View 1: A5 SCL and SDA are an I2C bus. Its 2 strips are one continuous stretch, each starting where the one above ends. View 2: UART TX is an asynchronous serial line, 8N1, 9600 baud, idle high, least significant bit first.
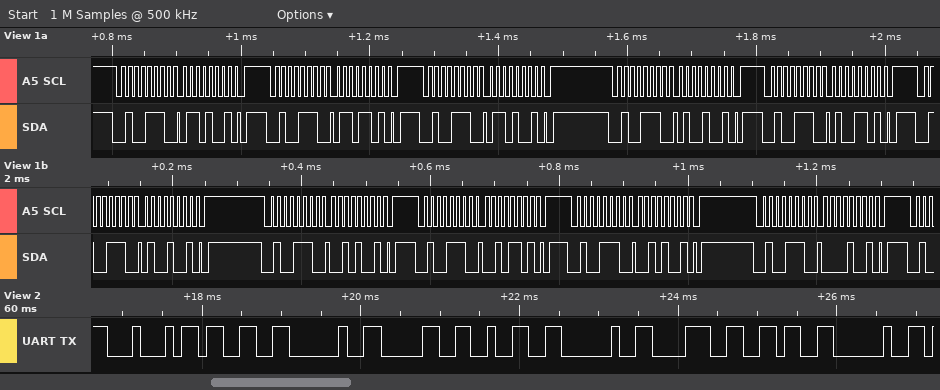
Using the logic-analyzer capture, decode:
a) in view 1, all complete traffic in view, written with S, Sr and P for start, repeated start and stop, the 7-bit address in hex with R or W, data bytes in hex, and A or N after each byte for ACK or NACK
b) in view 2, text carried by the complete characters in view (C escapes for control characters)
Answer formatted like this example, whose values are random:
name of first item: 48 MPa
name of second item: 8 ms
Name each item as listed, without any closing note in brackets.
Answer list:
in view 1, all complete traffic in view, written with S, Sr and P for start, repeated start and stop, the 7-bit address in hex with R or W, data bytes in hex, and A or N after each byte for ACK or NACK: S 27W A 69 A P S 27W A 6D A P S 27W A 69 A P S 27W A 49 A P S 27W A 4D A P S 27W A 49 A P S 27W A 29 A P S 27W A 2D A P S 27W A 29 A P S 27W A 09 A P
in view 2, text carried by the complete characters in view: "D3 02 86 "
